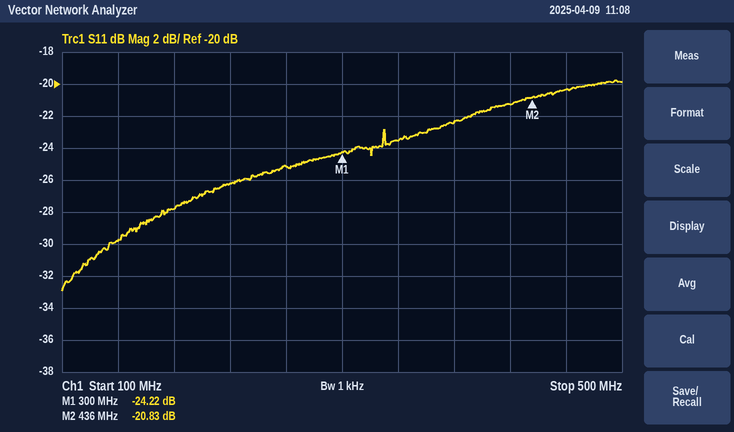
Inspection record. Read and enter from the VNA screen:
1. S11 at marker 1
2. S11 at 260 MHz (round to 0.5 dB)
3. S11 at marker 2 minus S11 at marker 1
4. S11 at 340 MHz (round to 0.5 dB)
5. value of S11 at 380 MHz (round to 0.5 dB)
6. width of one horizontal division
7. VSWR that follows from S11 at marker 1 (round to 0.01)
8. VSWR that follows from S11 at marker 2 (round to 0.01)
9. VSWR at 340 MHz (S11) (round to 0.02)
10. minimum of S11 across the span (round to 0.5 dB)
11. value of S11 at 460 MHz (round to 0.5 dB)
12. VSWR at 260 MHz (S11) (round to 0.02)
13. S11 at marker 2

-24.22 dB
-25.0 dB
3.39 dB
-23.5 dB
-22.5 dB
40 MHz
1.13
1.20
1.14
-33.0 dB
-20.5 dB
1.12
-20.83 dB
